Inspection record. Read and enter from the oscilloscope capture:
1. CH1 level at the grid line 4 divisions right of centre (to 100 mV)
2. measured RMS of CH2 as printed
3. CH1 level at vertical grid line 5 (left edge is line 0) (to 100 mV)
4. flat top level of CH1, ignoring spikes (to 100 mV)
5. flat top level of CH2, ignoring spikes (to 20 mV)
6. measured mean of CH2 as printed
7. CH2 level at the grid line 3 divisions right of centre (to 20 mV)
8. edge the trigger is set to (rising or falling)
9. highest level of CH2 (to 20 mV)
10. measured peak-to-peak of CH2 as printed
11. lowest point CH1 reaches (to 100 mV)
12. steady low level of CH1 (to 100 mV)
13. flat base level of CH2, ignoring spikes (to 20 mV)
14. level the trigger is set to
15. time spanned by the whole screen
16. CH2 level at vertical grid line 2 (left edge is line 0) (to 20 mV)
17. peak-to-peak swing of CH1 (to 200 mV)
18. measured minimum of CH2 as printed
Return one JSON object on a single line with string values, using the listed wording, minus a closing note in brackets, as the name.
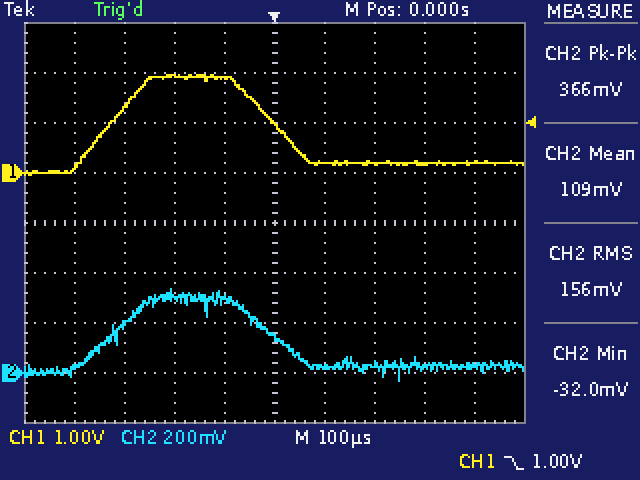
{"CH1 level at the grid line 4 divisions right of centre": "200 mV", "measured RMS of CH2 as printed": "156 mV", "CH1 level at vertical grid line 5 (left edge is line 0)": "1.0 V", "flat top level of CH1, ignoring spikes": "1.9 V", "flat top level of CH2, ignoring spikes": "300 mV", "measured mean of CH2 as printed": "109 mV", "CH2 level at the grid line 3 divisions right of centre": "20 mV", "edge the trigger is set to": "falling", "highest level of CH2": "340 mV", "measured peak-to-peak of CH2 as printed": "366 mV", "lowest point CH1 reaches": "0.0 V", "steady low level of CH1": "200 mV", "flat base level of CH2, ignoring spikes": "20 mV", "level the trigger is set to": "1.00 V", "time spanned by the whole screen": "1 ms", "CH2 level at vertical grid line 2 (left edge is line 0)": "200 mV", "peak-to-peak swing of CH1": "2.0 V", "measured minimum of CH2 as printed": "-32.0 mV"}
